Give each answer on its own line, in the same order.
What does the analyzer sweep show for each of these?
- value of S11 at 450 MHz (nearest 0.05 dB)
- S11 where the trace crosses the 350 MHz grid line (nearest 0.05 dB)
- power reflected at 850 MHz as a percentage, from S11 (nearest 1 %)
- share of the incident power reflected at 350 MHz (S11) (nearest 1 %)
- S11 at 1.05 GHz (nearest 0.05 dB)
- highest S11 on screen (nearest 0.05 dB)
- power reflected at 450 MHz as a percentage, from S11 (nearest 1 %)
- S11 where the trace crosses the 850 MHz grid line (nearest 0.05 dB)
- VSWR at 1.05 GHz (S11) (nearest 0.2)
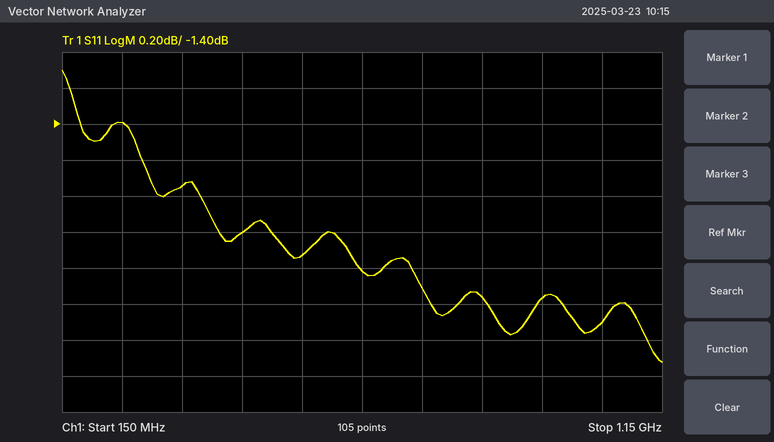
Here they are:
-2.00 dB
-1.75 dB
58 %
67 %
-2.50 dB
-1.10 dB
63 %
-2.35 dB
7.0
